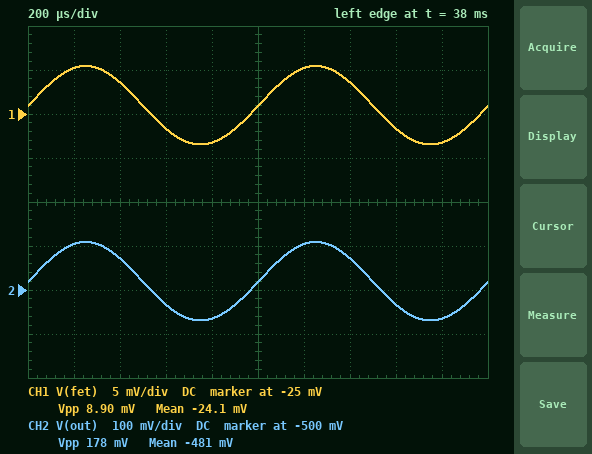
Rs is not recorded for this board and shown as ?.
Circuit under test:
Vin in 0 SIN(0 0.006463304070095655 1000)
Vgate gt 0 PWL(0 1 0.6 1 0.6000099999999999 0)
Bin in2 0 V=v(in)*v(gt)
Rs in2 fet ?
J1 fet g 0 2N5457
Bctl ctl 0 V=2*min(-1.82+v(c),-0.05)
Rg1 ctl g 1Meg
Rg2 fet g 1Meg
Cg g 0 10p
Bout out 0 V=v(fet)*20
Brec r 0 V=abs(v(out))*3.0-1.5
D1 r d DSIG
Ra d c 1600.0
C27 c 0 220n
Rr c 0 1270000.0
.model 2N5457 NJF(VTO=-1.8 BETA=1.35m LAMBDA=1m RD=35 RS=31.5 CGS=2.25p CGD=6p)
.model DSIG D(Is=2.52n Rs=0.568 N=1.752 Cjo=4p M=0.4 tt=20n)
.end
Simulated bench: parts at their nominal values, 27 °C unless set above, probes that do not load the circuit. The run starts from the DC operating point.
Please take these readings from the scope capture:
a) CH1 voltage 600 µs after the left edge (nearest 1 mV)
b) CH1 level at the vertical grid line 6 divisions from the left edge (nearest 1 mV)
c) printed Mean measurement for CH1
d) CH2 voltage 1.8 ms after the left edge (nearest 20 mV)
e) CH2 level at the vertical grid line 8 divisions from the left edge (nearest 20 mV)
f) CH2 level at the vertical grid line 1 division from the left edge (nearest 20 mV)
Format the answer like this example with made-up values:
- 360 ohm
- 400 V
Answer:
- -27 mV
- -20 mV
- -24.1 mV
- -560 mV
- -540 mV
- -400 mV
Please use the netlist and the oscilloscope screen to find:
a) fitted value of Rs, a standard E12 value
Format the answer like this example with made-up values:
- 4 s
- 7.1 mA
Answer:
- 18 kΩ
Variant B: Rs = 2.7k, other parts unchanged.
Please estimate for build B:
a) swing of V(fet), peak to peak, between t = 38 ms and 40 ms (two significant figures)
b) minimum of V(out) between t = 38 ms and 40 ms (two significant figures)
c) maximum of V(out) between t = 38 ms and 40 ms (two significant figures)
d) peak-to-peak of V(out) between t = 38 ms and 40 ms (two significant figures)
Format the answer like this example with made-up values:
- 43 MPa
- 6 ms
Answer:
- 13 mV
- -230 mV
- 31 mV
- 260 mV
